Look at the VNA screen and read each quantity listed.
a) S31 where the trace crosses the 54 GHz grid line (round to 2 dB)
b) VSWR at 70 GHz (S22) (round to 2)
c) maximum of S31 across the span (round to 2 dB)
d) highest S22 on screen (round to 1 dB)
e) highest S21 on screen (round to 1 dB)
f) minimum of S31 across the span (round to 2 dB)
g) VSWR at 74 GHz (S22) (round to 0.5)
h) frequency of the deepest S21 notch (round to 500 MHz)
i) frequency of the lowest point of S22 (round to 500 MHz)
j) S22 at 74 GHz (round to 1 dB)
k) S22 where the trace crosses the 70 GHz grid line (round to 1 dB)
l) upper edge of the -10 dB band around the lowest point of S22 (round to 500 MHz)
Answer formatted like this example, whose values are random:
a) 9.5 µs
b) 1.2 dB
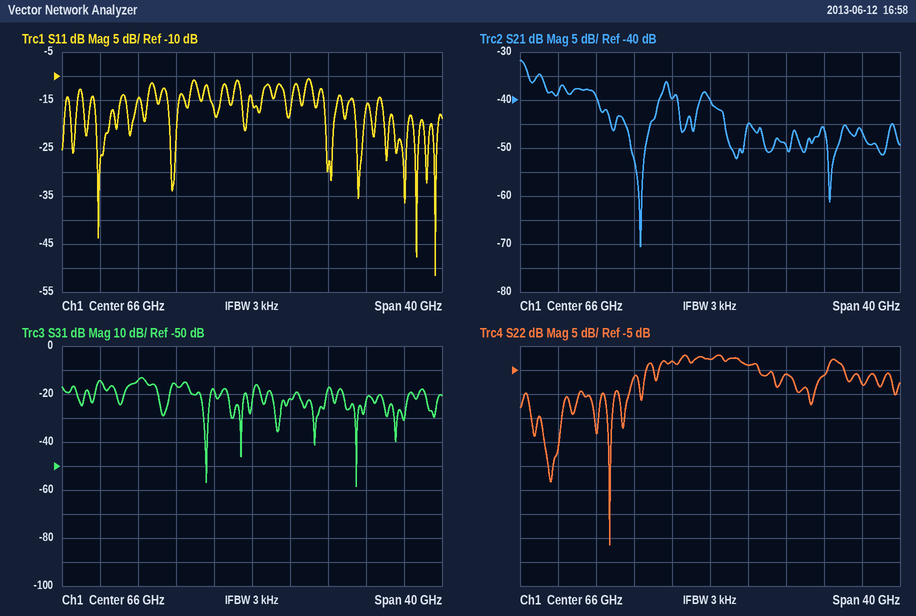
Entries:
a) -14 dB
b) 4
c) -14 dB
d) -2 dB
e) -32 dB
f) -58 dB
g) 3.0
h) 58.5 GHz
i) 55.5 GHz
j) -6 dB
k) -4 dB
l) 56.0 GHz
